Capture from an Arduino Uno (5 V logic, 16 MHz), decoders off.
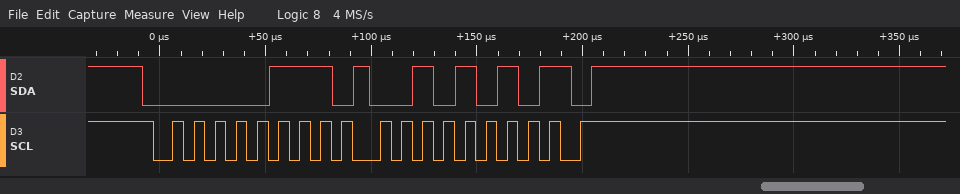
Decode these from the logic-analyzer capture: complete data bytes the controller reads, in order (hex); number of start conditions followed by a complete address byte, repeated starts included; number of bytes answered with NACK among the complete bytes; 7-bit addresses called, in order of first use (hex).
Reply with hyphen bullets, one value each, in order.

- 2A
- 1
- 1
- 0x03
